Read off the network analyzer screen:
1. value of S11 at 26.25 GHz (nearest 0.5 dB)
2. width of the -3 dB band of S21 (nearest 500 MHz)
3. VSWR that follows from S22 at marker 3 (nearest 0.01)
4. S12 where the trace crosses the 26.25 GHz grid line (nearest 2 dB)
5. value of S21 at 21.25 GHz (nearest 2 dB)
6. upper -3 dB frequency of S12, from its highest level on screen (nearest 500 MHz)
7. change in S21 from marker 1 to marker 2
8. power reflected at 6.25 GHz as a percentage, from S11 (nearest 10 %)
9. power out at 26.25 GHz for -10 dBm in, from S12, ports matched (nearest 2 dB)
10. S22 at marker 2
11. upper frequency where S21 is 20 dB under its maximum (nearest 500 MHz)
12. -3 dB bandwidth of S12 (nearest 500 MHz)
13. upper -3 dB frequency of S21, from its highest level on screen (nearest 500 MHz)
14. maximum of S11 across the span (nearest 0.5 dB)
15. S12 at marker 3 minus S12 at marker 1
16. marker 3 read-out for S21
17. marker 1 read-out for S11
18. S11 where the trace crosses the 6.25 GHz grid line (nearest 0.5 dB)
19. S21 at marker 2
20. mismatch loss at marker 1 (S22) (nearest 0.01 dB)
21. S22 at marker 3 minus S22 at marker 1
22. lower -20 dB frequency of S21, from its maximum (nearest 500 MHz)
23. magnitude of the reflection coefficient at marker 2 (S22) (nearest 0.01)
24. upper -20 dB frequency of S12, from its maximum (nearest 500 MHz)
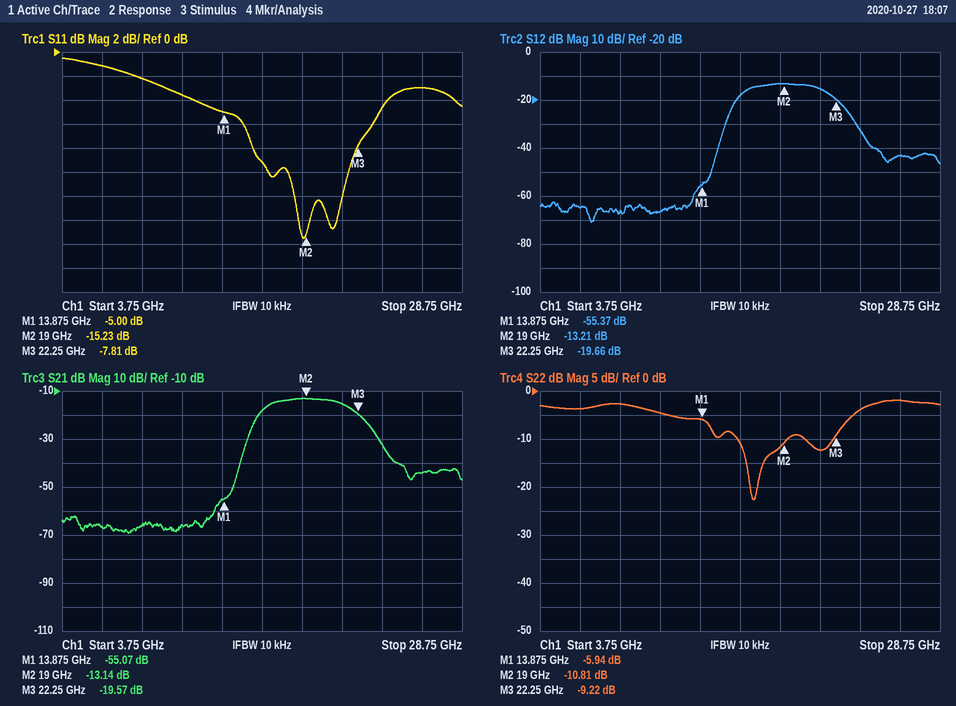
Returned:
-3.0 dB
5.0 GHz
2.06
-44 dB
-16 dB
21.5 GHz
41.93 dB
80 %
-54 dBm
-10.81 dB
24.0 GHz
5.0 GHz
21.5 GHz
-0.5 dB
35.71 dB
-19.57 dB
-5.00 dB
-1.0 dB
-13.14 dB
1.28 dB
-3.28 dB
15.0 GHz
0.29
24.0 GHz
